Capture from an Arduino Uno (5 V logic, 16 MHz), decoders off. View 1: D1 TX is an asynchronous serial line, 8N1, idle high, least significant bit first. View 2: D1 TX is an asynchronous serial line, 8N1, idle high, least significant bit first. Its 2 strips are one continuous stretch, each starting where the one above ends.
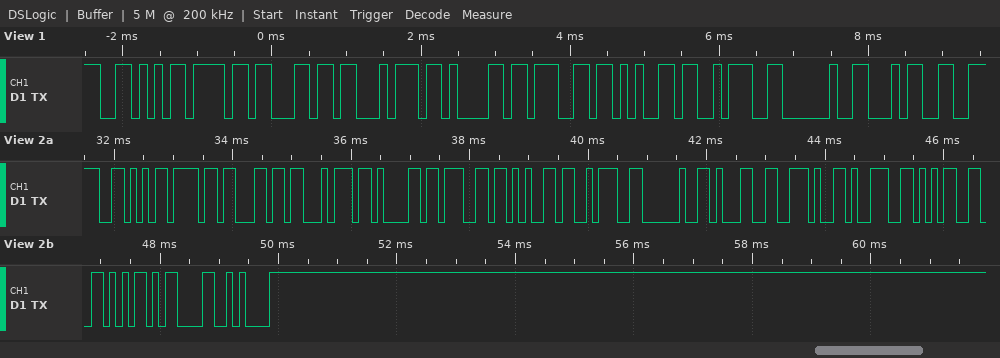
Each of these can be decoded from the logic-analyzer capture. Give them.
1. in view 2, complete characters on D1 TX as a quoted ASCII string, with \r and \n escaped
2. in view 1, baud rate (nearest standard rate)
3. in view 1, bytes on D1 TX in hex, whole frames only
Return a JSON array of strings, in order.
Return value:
["\"Voltage: 1.95V\\r\\n\"", "9600 baud", "0x56 0x6F 0x6C 0x74 0x61 0x67 0x65 0x3A 0x20 0x34"]
